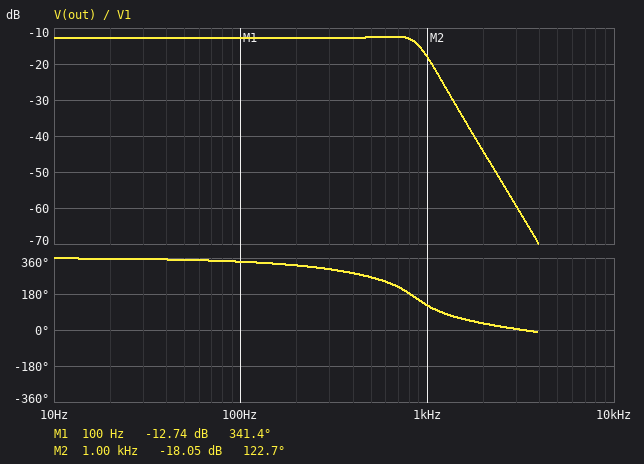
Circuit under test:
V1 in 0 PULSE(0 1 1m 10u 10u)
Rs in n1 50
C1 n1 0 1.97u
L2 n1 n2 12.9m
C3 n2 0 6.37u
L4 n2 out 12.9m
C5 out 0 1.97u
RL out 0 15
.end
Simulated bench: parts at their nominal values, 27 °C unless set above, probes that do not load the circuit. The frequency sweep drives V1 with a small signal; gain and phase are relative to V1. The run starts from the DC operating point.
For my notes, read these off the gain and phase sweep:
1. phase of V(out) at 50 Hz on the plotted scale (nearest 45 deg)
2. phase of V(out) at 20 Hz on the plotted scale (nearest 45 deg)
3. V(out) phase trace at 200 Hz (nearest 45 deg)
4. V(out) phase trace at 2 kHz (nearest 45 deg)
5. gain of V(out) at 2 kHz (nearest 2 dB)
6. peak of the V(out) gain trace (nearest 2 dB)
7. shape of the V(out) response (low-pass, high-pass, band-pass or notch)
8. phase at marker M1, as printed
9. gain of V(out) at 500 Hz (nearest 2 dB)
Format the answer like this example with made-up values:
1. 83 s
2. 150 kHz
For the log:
1. 360 deg
2. 360 deg
3. 315 deg
4. 45 deg
5. -44 dB
6. -12 dB
7. low-pass
8. 341.4 deg
9. -12 dB
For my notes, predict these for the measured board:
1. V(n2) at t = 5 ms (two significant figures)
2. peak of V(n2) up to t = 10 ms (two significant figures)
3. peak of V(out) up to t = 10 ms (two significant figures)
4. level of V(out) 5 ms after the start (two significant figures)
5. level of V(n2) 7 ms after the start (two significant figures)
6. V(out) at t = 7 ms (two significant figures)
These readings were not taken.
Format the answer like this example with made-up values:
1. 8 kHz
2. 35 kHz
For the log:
1. 230 mV
2. 560 mV
3. 260 mV
4. 230 mV
5. 230 mV
6. 230 mV
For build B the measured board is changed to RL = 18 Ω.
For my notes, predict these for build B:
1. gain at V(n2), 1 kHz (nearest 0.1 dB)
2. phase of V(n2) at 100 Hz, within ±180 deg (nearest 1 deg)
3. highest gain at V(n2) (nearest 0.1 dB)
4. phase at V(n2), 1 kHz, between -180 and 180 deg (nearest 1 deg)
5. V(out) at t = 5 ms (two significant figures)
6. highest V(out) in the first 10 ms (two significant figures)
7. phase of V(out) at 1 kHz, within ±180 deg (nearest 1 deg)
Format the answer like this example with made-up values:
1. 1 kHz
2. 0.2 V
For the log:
1. -3.5 dB
2. 6 deg
3. -0.6 dB
4. -146 deg
5. 260 mV
6. 300 mV
7. 124 deg
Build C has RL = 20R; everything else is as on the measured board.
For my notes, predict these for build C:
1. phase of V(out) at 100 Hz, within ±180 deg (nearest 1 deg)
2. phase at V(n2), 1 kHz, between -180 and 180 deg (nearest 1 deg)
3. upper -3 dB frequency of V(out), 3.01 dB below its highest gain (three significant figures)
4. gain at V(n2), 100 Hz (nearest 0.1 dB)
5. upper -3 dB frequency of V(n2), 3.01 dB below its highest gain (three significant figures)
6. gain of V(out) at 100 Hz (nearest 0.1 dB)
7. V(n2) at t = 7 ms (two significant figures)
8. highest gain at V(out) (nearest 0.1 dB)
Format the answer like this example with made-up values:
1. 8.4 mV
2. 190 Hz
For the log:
1. -19 deg
2. -145 deg
3. 929 Hz
4. -10.3 dB
5. 1.01 kHz
6. -10.9 dB
7. 290 mV
8. -10.6 dB
